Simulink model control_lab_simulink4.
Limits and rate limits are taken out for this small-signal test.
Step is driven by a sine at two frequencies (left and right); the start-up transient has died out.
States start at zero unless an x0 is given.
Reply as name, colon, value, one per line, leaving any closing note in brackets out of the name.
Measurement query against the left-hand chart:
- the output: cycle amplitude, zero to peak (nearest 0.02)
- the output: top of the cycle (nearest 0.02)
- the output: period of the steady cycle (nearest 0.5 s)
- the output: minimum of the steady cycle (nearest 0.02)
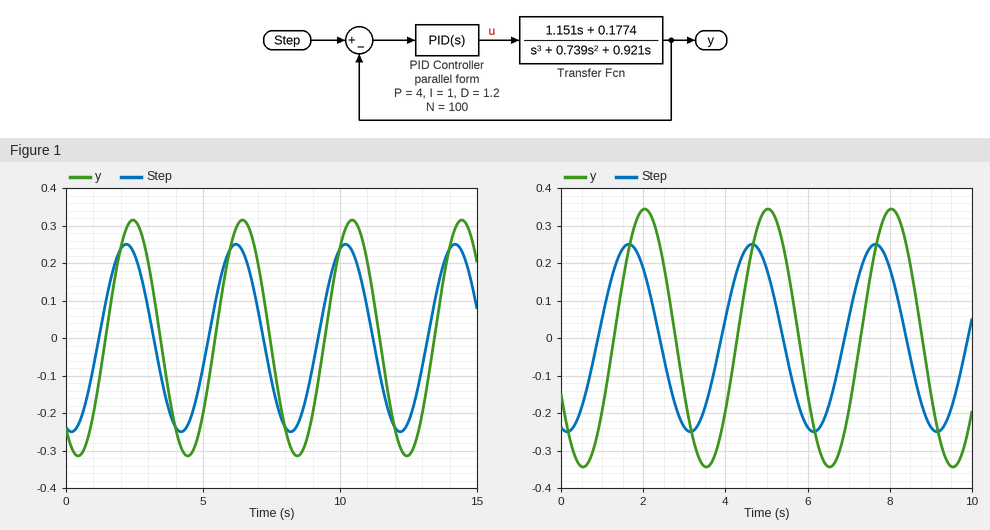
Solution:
the output: cycle amplitude, zero to peak: 0.32
the output: top of the cycle: 0.32
the output: period of the steady cycle: 4.0 s
the output: minimum of the steady cycle: -0.32
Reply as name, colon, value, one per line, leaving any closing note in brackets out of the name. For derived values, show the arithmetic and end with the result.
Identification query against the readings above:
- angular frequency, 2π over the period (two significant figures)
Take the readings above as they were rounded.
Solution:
angular frequency, 2π over the period: 2π / 4 = 1.6 rad/s
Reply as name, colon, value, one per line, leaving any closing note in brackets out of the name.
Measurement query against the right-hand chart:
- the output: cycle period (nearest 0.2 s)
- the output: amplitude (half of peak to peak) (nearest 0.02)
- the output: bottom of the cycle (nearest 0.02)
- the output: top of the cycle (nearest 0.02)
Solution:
the output: cycle period: 3.0 s
the output: amplitude (half of peak to peak): 0.34
the output: bottom of the cycle: -0.34
the output: top of the cycle: 0.34
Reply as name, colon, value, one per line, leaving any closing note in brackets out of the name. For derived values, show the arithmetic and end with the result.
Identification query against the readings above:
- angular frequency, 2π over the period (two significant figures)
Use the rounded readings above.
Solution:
angular frequency, 2π over the period: 2π / 3 = 2.1 rad/s
